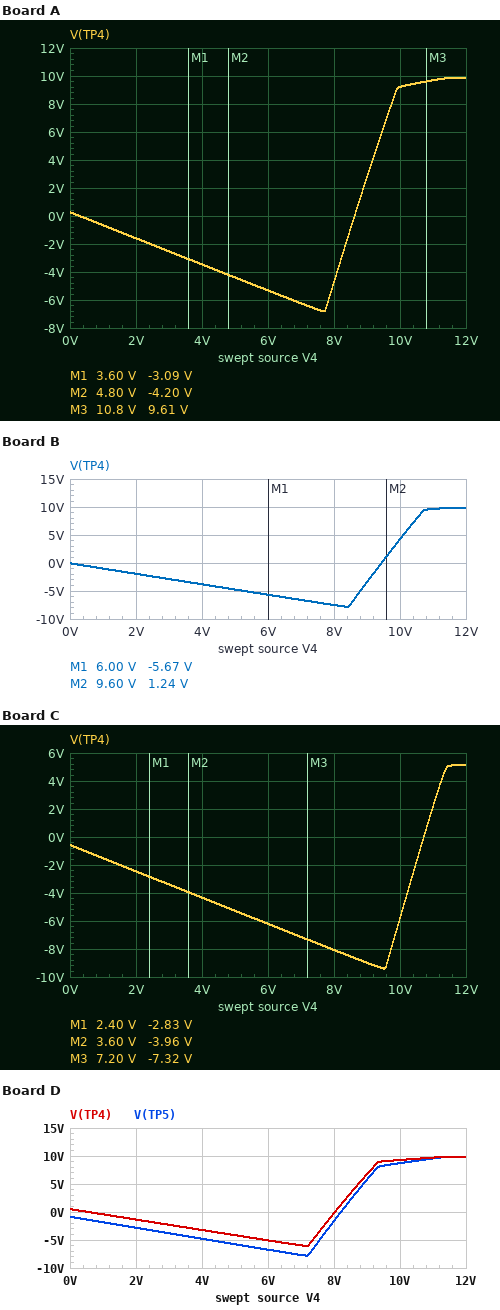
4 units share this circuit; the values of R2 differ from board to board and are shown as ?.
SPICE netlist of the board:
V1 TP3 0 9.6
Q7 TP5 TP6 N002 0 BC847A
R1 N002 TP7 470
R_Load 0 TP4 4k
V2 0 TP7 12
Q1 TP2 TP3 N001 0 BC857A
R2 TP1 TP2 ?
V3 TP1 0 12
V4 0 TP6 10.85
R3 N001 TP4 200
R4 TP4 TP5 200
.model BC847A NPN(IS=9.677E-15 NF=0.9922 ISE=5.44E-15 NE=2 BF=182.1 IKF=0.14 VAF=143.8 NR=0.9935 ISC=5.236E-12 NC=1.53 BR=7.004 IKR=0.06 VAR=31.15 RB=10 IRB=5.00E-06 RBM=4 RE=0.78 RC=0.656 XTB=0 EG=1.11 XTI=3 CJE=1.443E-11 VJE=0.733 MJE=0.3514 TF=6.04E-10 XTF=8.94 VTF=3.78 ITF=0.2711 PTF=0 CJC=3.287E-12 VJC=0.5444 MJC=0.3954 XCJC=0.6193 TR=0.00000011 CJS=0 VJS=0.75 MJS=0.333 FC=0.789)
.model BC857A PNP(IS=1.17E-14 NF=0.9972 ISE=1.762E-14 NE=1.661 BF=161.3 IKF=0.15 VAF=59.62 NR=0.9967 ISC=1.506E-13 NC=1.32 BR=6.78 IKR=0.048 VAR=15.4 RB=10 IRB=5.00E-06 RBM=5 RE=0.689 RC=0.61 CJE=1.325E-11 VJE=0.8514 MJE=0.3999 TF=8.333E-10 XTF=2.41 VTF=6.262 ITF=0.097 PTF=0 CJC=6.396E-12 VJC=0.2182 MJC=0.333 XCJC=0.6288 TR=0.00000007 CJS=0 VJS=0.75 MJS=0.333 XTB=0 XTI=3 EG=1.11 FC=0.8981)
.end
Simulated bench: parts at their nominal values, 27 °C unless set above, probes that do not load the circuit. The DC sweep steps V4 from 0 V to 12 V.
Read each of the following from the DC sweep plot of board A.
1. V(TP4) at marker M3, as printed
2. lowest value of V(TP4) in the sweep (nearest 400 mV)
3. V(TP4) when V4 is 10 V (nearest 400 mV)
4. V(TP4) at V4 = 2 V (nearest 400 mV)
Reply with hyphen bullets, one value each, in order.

- 9.61 V
- -6.8 V
- 9.2 V
- -1.6 V
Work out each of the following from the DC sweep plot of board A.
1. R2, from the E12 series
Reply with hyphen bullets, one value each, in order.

- 270 Ω
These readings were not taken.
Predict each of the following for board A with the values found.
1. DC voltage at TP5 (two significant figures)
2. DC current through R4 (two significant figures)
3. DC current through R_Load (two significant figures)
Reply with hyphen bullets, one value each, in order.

- 9.4 V
- 1.1 mA
- 2.4 mA
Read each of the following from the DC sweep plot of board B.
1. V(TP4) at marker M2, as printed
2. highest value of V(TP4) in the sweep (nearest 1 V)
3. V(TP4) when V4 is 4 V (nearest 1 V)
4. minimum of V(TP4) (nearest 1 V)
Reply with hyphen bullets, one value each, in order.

- 1.24 V
- 10 V
- -4 V
- -8 V
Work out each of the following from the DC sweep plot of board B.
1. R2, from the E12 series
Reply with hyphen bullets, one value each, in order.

- 390 Ω
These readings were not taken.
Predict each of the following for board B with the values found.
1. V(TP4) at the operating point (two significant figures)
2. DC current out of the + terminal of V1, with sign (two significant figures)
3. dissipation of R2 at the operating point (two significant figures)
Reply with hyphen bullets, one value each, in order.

- 9.6 V
- -910 µA
- 7.4 mW
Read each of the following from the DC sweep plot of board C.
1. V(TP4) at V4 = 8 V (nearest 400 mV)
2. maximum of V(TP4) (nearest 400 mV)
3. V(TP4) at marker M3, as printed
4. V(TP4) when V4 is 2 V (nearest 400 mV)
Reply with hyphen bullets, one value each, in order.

- -8.0 V
- 5.2 V
- -7.32 V
- -2.4 V
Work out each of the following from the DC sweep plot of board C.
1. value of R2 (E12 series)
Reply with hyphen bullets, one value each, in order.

- 1.2 kΩ
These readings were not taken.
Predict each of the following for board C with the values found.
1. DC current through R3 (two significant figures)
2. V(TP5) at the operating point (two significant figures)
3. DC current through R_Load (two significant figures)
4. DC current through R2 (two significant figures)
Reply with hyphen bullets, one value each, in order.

- 1.3 mA
- 800 mV
- 250 µA
- 1.5 mA
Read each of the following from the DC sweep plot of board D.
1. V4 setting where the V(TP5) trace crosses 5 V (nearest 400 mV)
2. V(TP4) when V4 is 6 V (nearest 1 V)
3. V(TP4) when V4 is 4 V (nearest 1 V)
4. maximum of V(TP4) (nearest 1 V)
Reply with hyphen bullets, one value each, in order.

- 8.8 V
- -5 V
- -3 V
- 10 V
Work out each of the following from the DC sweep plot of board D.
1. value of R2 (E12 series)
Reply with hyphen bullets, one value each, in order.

- 220 Ω
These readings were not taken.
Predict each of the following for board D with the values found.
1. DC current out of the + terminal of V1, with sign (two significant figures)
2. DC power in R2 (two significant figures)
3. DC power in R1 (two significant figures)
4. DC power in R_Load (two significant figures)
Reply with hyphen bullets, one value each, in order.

- -4.0 mA
- 12 mW
- 530 µW
- 23 mW
